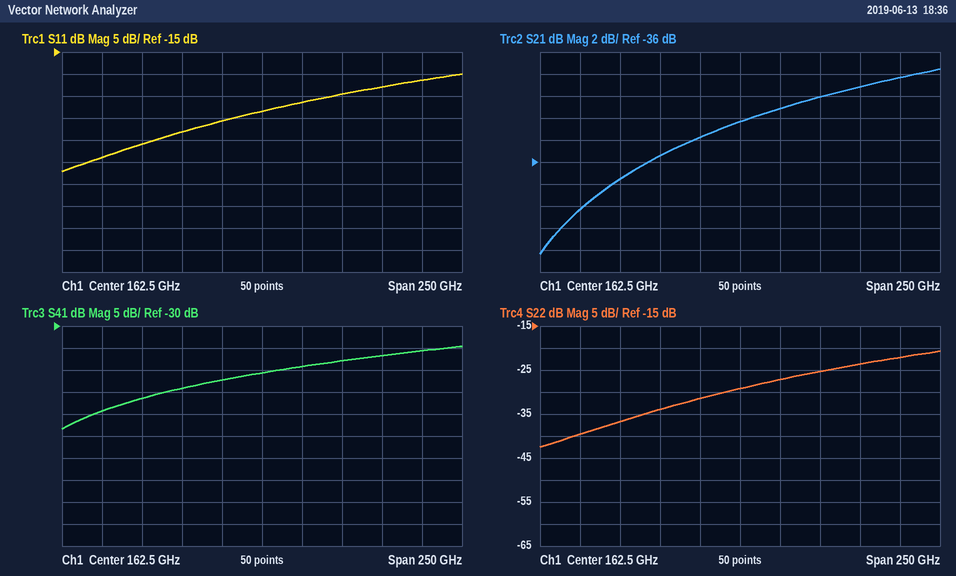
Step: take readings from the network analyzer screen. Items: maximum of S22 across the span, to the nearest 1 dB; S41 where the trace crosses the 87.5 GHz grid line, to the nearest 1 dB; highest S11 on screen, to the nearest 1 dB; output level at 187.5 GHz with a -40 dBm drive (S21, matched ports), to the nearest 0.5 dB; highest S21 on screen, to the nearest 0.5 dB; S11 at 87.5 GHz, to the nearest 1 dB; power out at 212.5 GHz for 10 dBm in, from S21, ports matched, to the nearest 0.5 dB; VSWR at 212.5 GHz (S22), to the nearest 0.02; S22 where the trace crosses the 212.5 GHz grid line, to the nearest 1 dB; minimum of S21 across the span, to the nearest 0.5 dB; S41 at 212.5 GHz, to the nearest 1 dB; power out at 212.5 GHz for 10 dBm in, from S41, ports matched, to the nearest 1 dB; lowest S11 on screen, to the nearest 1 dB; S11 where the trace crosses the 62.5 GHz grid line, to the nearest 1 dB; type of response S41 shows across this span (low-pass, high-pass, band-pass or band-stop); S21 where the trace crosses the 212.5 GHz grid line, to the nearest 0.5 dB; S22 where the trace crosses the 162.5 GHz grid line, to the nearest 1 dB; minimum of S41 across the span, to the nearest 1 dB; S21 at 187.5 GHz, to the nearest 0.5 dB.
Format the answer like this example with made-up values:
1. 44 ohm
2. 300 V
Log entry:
1. -21 dB
2. -46 dB
3. -20 dB
4. -71.0 dBm
5. -27.5 dB
6. -36 dB
7. -20.0 dBm
8. 1.12
9. -25 dB
10. -44.5 dB
11. -38 dB
12. -28 dBm
13. -42 dB
14. -39 dB
15. high-pass
16. -30.0 dB
17. -29 dB
18. -53 dB
19. -31.0 dB
